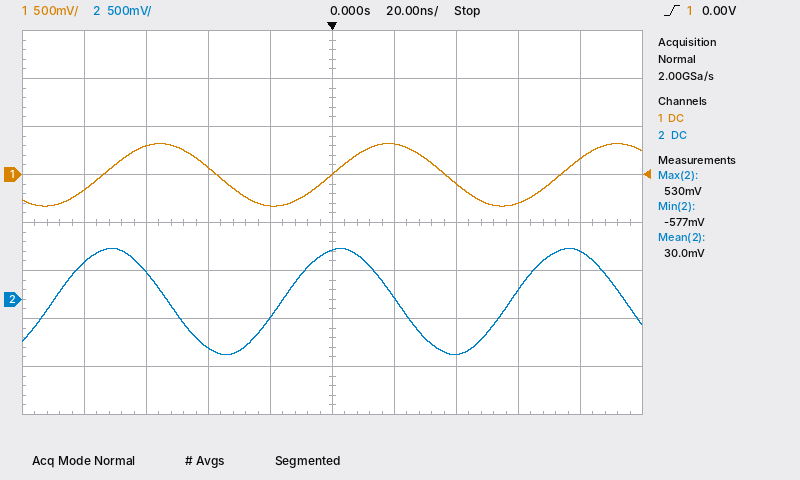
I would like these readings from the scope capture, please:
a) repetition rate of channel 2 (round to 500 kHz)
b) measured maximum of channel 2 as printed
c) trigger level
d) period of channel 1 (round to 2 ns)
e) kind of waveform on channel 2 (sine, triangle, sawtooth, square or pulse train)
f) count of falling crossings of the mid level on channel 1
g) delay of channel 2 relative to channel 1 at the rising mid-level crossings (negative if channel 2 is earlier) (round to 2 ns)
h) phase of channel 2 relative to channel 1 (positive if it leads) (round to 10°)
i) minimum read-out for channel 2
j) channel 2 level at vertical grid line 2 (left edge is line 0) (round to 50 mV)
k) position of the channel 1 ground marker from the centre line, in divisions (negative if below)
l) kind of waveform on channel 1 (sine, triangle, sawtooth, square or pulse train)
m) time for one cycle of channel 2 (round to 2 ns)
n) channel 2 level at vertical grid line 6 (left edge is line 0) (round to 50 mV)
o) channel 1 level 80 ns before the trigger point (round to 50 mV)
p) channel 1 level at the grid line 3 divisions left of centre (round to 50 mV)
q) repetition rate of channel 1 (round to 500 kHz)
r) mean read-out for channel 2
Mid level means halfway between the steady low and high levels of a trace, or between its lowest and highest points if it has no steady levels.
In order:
13.5 MHz
530 mV
0.00 V
74 ns
sine
2
-16 ns
+80°
-577 mV
300 mV
+1.0 div
sine
74 ns
0 mV
-150 mV
300 mV
13.5 MHz
30.0 mV
